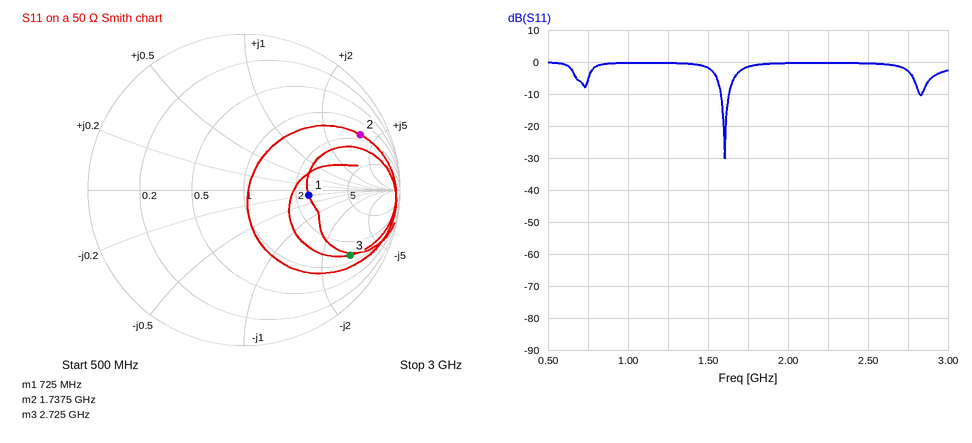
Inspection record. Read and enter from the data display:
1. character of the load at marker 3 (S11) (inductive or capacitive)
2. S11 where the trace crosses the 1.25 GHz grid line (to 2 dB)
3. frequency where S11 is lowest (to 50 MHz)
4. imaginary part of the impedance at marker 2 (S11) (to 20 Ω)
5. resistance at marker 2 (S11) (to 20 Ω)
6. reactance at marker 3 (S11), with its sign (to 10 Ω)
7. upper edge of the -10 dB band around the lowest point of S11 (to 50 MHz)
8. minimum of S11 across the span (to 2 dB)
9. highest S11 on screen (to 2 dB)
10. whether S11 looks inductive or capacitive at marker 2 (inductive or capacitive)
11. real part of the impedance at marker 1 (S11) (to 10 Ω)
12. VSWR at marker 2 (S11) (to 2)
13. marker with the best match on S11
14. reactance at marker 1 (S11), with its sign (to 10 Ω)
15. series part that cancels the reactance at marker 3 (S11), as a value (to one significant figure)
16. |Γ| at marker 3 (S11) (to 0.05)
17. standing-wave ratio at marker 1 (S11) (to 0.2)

capacitive
0 dB
1.60 GHz
+180 Ω
80 Ω
-150 Ω
1.65 GHz
-30 dB
0 dB
inductive
120 Ω
10
marker 1
-10 Ω
9 nH
0.80
2.4
